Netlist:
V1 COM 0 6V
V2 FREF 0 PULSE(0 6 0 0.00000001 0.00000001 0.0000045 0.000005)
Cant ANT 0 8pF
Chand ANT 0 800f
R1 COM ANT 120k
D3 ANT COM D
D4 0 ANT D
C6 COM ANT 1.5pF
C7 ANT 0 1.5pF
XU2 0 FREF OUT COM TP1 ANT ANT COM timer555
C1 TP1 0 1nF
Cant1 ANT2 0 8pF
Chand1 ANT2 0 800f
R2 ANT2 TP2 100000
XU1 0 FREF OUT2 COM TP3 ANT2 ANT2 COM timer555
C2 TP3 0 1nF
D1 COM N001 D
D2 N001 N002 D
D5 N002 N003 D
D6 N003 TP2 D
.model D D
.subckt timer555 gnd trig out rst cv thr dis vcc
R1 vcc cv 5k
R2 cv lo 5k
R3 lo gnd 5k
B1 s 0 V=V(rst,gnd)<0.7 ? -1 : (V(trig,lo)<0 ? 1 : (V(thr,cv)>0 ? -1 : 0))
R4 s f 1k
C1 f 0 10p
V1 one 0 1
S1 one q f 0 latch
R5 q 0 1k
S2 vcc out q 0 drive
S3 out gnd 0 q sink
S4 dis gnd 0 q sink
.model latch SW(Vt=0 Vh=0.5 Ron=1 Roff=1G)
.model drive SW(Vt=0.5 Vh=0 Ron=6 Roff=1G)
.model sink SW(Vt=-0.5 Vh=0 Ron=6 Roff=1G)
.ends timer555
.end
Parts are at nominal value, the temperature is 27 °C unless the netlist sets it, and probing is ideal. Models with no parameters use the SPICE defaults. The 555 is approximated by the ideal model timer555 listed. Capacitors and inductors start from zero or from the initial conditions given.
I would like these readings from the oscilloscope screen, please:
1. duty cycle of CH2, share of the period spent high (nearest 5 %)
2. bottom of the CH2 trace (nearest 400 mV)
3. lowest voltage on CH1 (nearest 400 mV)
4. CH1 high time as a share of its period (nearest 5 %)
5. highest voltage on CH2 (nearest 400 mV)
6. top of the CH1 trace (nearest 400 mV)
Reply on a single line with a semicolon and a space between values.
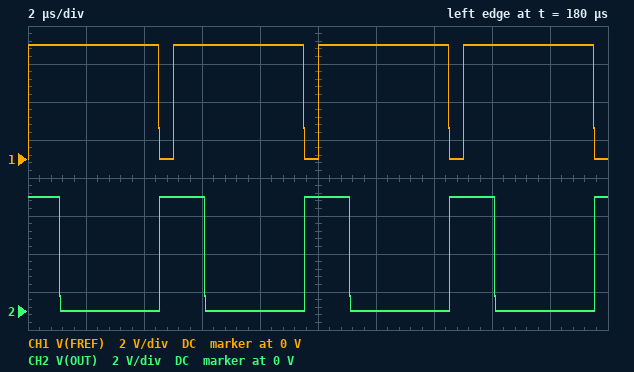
30 %; 0 V; 0 V; 90 %; 6.0 V; 6.0 V
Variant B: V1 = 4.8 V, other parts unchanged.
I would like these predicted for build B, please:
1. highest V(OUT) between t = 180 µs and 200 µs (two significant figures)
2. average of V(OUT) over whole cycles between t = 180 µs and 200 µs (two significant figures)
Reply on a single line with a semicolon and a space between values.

4.8 V; 1.5 V
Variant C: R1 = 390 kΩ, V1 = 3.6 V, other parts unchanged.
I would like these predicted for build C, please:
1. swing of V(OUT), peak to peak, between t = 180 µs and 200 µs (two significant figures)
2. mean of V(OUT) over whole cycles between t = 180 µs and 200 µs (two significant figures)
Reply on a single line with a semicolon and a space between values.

3.6 V; 2.0 V
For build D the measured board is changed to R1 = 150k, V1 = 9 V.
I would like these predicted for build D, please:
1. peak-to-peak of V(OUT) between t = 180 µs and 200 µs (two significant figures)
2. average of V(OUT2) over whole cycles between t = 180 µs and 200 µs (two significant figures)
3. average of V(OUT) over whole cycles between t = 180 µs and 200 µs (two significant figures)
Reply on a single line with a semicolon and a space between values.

9.0 V; 3.4 V; 3.5 V
